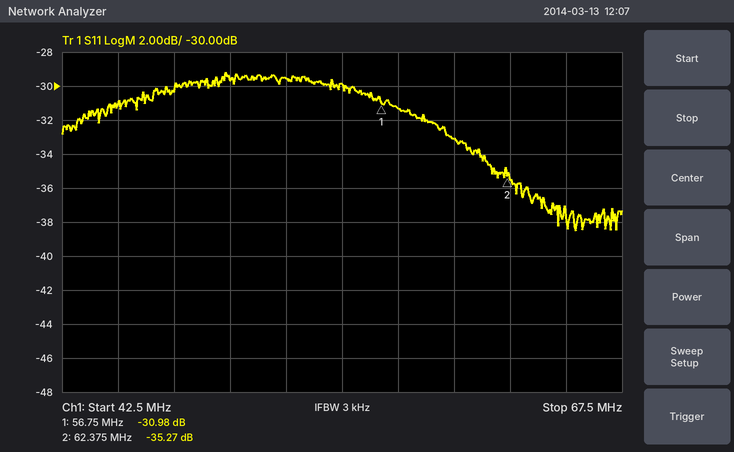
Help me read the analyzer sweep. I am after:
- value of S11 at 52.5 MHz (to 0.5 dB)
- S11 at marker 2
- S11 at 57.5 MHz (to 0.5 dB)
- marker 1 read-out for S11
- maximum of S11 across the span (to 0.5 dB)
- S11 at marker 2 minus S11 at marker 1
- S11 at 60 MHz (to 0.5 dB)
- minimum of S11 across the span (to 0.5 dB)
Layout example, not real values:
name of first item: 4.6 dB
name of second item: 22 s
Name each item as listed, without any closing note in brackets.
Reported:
value of S11 at 52.5 MHz: -29.5 dB
S11 at marker 2: -35.27 dB
S11 at 57.5 MHz: -31.5 dB
marker 1 read-out for S11: -30.98 dB
maximum of S11 across the span: -29.0 dB
S11 at marker 2 minus S11 at marker 1: -4.29 dB
S11 at 60 MHz: -33.0 dB
minimum of S11 across the span: -38.5 dB
